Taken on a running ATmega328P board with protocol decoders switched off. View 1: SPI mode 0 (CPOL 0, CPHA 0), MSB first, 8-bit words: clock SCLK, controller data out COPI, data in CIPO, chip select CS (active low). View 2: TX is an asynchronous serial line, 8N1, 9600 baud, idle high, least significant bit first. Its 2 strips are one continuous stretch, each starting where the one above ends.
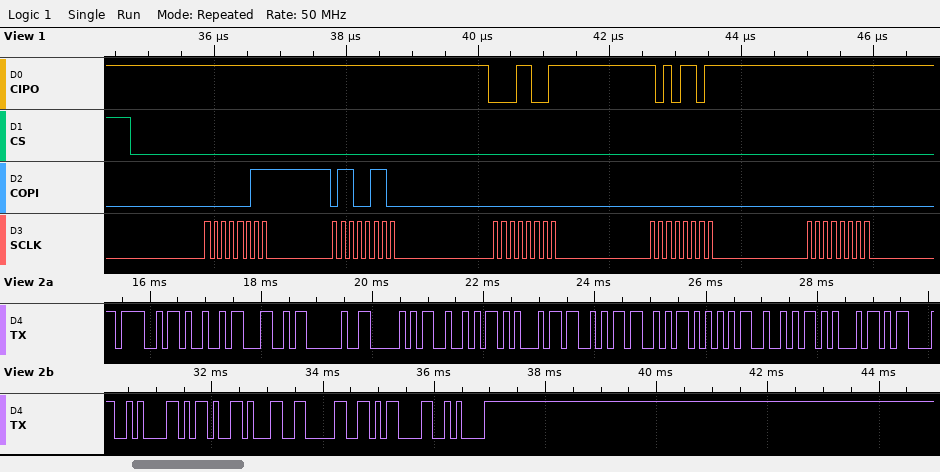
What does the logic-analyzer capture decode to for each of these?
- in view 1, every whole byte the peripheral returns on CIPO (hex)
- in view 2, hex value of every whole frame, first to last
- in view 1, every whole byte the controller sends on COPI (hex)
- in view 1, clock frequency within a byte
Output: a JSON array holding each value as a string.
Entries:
["FF FF 19 AD FF", "0x4F 0x49 0x4C 0x20 0x50 0x52 0x45 0x53 0x53 0x55 0x52 0x45 0x0D 0x0A 0x2D 0x31 0x30 0x0D 0x0A", "03 66 00 00 00", "8 MHz"]
